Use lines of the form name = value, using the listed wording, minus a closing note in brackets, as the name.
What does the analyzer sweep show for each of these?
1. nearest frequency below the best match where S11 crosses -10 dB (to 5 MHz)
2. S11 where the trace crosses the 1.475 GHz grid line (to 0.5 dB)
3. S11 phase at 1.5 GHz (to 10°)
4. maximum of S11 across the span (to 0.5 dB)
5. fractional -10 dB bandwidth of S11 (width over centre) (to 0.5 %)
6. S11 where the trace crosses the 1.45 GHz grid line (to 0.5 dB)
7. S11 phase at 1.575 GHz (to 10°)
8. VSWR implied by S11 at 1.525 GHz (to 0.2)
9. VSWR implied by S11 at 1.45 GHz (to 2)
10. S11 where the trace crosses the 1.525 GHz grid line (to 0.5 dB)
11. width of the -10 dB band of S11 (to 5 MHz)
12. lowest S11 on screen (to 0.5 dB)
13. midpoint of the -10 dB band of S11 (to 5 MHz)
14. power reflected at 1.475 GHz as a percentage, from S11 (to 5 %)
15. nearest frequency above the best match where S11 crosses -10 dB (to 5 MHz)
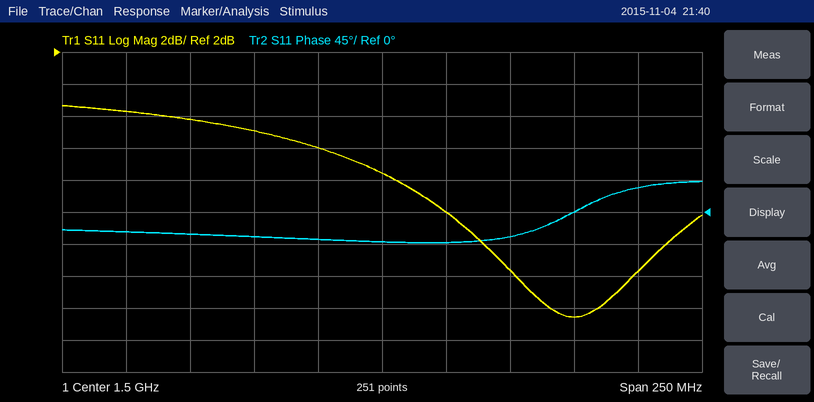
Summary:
nearest frequency below the best match where S11 crosses -10 dB = 1.540 GHz
S11 where the trace crosses the 1.475 GHz grid line = -4.0 dB
S11 phase at 1.5 GHz = -40°
maximum of S11 across the span = -1.5 dB
fractional -10 dB bandwidth of S11 (width over centre) = 4.5 %
S11 where the trace crosses the 1.45 GHz grid line = -3.0 dB
S11 phase at 1.575 GHz = 0°
VSWR implied by S11 at 1.525 GHz = 2.4
VSWR implied by S11 at 1.45 GHz = 6
S11 where the trace crosses the 1.525 GHz grid line = -8.0 dB
width of the -10 dB band of S11 = 70 MHz
lowest S11 on screen = -14.5 dB
midpoint of the -10 dB band of S11 = 1.575 GHz
power reflected at 1.475 GHz as a percentage, from S11 = 40 %
nearest frequency above the best match where S11 crosses -10 dB = 1.610 GHz
